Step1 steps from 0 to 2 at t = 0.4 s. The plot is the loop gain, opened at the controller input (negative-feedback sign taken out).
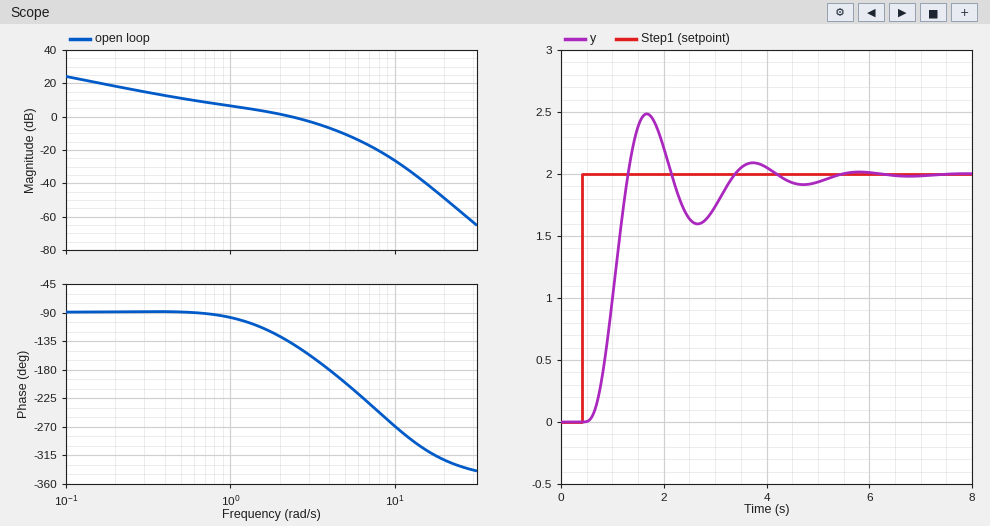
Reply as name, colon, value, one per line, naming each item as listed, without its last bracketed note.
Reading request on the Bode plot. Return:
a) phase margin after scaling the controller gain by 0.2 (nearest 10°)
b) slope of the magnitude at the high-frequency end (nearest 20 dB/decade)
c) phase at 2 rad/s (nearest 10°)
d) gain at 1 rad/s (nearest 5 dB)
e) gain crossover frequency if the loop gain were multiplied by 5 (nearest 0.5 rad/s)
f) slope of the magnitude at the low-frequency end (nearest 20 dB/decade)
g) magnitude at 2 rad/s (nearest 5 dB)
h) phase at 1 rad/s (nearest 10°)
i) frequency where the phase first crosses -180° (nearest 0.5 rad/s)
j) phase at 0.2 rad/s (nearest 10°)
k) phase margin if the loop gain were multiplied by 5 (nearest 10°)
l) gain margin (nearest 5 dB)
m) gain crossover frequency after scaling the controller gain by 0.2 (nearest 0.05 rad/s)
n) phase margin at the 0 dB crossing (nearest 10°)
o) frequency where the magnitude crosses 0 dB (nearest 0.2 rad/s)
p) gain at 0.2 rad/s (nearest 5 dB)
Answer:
phase margin after scaling the controller gain by 0.2: 90°
slope of the magnitude at the high-frequency end: -80 dB/decade
phase at 2 rad/s: -130°
gain at 1 rad/s: 5 dB
gain crossover frequency if the loop gain were multiplied by 5: 6.0 rad/s
slope of the magnitude at the low-frequency end: -20 dB/decade
magnitude at 2 rad/s: 0 dB
phase at 1 rad/s: -100°
frequency where the phase first crosses -180°: 4.0 rad/s
phase at 0.2 rad/s: -90°
phase margin if the loop gain were multiplied by 5: -40°
gain margin: 5 dB
gain crossover frequency after scaling the controller gain by 0.2: 0.35 rad/s
phase margin at the 0 dB crossing: 40°
frequency where the magnitude crosses 0 dB: 2.4 rad/s
gain at 0.2 rad/s: 20 dB
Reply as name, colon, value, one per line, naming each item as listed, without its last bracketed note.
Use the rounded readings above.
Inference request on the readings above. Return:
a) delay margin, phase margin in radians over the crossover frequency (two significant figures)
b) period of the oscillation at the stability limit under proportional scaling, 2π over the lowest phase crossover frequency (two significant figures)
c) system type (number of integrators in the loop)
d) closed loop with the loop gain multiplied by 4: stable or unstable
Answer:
delay margin, phase margin in radians over the crossover frequency: 0.29 s
period of the oscillation at the stability limit under proportional scaling, 2π over the lowest phase crossover frequency: 1.6 s
system type: 1
closed loop with the loop gain multiplied by 4: stable or unstable: unstable
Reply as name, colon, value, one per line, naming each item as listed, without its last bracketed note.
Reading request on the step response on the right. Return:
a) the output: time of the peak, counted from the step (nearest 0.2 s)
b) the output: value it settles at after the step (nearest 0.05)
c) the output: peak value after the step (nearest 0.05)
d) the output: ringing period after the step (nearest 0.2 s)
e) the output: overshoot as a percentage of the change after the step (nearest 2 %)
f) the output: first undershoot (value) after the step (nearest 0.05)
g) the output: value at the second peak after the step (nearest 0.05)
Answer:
the output: time of the peak, counted from the step: 1.2 s
the output: value it settles at after the step: 2.00
the output: peak value after the step: 2.50
the output: ringing period after the step: 2.0 s
the output: overshoot as a percentage of the change after the step: 24 %
the output: first undershoot (value) after the step: 1.60
the output: value at the second peak after the step: 2.10
